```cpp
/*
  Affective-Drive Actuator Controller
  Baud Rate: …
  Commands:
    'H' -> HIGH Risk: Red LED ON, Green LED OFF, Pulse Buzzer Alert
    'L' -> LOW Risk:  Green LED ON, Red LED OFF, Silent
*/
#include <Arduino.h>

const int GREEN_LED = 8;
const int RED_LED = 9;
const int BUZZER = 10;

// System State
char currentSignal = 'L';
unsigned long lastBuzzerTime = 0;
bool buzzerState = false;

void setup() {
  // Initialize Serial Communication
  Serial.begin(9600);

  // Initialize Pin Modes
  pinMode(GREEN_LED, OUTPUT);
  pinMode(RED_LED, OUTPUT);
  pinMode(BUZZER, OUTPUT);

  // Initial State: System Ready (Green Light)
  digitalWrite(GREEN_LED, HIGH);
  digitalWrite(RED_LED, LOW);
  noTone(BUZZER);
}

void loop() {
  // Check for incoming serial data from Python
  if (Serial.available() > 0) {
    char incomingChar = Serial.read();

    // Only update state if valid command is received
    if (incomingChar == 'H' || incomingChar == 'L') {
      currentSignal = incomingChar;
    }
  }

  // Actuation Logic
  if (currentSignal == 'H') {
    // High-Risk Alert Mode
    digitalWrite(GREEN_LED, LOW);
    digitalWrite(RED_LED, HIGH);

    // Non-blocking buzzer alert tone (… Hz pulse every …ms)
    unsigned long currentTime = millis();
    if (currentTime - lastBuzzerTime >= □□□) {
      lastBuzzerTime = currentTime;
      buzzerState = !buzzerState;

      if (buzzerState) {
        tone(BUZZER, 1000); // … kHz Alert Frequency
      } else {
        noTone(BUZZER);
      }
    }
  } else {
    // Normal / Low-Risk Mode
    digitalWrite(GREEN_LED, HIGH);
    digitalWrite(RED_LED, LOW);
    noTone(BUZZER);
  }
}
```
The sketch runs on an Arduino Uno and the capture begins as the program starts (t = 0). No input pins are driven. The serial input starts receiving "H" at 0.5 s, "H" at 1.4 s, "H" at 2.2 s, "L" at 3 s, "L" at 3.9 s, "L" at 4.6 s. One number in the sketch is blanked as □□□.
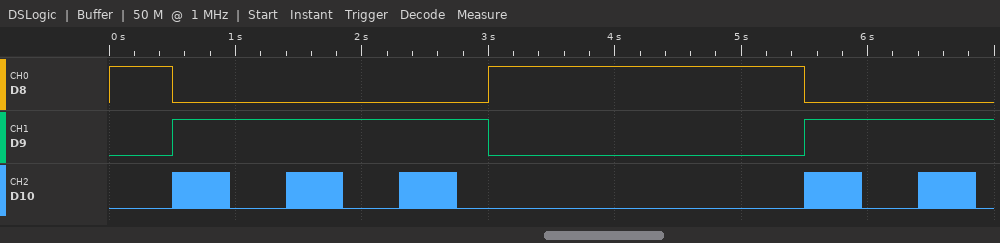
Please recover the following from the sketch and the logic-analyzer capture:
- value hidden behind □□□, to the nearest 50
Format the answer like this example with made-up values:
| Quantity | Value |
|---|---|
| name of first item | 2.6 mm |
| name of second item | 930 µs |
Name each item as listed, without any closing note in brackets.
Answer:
| Quantity | Value |
|---|---|
| value hidden behind □□□, to the nearest 50 | 450 |
